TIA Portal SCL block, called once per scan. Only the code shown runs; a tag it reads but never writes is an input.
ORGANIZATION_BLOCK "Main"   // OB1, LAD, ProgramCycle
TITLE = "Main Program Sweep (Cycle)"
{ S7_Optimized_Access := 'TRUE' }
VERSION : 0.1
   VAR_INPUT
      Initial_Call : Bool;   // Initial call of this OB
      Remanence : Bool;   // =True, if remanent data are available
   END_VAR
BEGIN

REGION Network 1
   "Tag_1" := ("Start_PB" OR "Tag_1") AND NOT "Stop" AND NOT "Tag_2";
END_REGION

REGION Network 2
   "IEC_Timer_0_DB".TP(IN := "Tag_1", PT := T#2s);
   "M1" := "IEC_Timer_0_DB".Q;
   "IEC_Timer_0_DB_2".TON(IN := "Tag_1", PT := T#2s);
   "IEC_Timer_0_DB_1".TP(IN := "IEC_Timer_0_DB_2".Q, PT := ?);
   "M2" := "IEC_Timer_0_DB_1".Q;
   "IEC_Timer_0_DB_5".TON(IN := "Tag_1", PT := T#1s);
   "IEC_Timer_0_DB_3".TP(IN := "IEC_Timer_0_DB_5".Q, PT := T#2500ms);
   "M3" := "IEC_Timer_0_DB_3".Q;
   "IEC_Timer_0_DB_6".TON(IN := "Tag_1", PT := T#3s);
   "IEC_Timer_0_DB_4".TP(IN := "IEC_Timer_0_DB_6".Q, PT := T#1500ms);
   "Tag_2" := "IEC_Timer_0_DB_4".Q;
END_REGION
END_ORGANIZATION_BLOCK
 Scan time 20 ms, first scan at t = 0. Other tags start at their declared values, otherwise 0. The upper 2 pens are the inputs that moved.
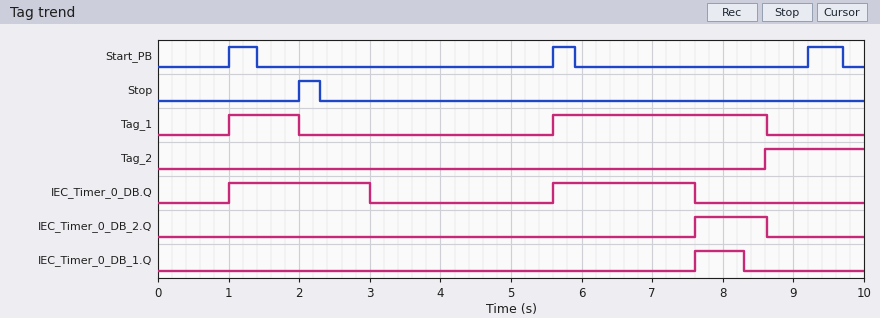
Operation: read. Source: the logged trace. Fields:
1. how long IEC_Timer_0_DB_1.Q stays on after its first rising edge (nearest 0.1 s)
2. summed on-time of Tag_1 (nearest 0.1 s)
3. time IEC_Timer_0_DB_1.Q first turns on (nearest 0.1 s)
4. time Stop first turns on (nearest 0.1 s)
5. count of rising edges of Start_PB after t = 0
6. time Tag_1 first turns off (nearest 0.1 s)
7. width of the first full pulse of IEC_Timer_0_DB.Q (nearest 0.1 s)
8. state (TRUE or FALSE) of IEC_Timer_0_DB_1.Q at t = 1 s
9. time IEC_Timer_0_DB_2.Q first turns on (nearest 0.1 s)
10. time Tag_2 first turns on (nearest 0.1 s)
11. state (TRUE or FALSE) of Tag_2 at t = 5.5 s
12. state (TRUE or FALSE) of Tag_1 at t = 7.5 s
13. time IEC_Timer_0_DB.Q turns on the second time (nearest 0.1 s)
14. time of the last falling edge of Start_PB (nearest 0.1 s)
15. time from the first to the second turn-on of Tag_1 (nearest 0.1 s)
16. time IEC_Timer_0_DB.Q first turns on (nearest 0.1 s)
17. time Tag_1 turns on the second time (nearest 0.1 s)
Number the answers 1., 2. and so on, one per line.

1. 0.7 s
2. 4.0 s
3. 7.6 s
4. 2.0 s
5. 3
6. 2.0 s
7. 2.0 s
8. FALSE
9. 7.6 s
10. 8.6 s
11. FALSE
12. TRUE
13. 5.6 s
14. 9.7 s
15. 4.6 s
16. 1.0 s
17. 5.6 s
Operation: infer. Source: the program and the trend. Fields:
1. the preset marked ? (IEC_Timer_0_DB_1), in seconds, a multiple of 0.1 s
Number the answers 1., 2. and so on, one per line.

1. 0.7 s
